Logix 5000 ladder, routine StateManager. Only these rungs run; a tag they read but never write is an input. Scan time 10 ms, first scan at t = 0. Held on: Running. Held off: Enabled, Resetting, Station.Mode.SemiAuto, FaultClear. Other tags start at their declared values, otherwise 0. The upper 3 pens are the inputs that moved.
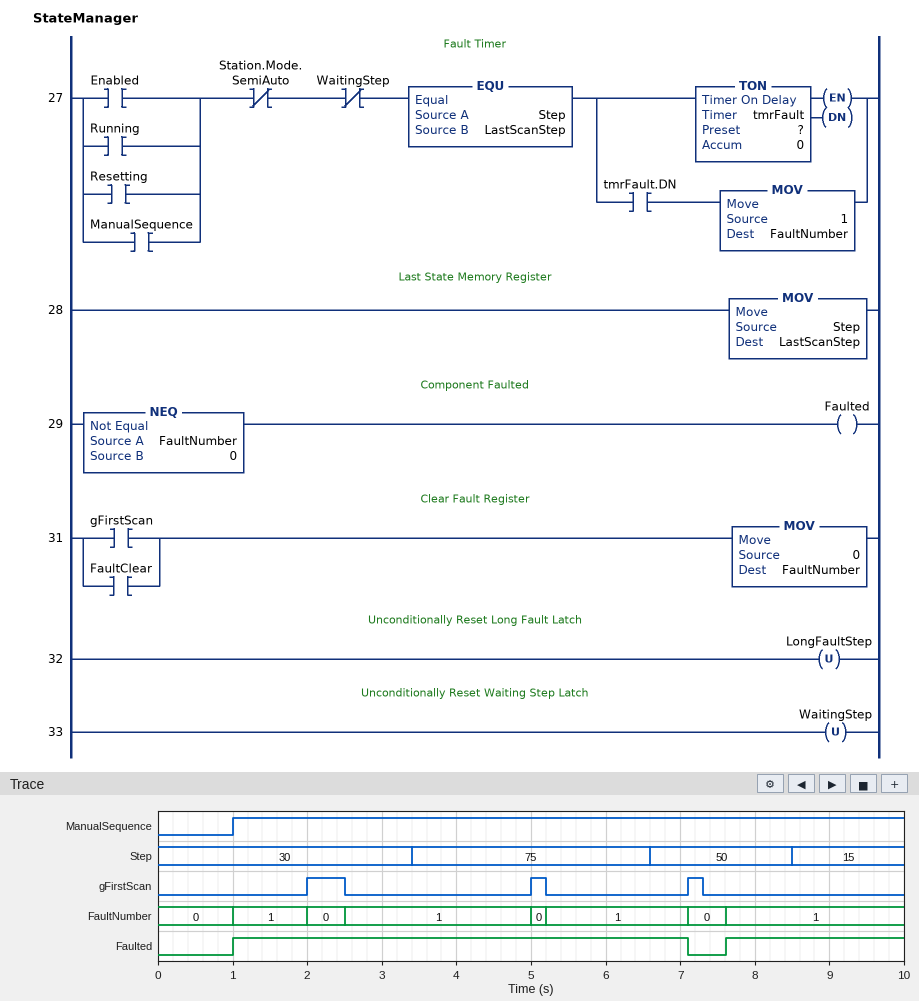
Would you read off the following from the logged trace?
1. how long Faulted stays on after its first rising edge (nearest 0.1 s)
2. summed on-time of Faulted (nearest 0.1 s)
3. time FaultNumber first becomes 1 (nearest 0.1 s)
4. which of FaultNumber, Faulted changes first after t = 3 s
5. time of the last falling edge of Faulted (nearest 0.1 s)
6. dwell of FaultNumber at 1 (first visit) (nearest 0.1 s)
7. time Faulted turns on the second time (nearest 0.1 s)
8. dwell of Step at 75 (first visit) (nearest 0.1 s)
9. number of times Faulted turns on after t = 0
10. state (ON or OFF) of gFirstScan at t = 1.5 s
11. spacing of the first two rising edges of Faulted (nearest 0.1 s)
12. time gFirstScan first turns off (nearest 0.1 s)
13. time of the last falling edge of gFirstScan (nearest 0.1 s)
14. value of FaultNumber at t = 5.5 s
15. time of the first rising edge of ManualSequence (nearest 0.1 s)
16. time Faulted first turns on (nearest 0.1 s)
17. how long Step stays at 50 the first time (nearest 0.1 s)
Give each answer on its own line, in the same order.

6.1 s
8.5 s
1.0 s
FaultNumber
7.1 s
1.0 s
7.6 s
3.2 s
2
OFF
6.6 s
2.5 s
7.3 s
1
1.0 s
1.0 s
1.9 s
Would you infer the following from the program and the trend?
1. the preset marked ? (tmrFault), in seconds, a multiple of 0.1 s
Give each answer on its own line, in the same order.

1.0 s
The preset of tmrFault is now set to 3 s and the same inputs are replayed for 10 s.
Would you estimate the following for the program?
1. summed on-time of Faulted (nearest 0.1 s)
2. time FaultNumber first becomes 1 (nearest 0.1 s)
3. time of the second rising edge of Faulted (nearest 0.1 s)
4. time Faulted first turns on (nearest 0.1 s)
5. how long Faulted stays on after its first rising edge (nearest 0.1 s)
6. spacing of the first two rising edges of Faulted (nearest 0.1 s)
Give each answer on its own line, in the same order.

2.7 s
3.0 s
6.4 s
3.0 s
2.0 s
3.4 s
